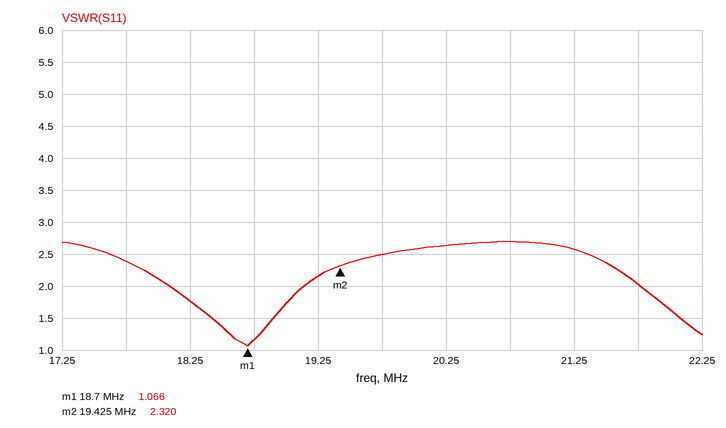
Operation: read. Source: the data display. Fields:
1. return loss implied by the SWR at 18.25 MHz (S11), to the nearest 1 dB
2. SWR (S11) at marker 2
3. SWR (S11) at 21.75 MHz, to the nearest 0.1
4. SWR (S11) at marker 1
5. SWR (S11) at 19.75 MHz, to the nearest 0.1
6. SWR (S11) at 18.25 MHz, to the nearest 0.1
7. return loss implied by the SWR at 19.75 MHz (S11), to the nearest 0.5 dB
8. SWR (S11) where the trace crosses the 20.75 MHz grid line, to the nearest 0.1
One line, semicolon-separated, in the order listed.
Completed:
11 dB; 2.320; 2.0; 1.066; 2.5; 1.8; 7.5 dB; 2.7
